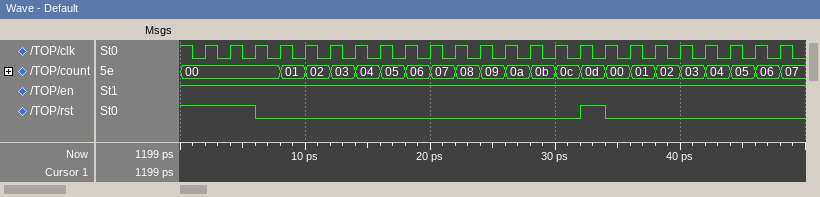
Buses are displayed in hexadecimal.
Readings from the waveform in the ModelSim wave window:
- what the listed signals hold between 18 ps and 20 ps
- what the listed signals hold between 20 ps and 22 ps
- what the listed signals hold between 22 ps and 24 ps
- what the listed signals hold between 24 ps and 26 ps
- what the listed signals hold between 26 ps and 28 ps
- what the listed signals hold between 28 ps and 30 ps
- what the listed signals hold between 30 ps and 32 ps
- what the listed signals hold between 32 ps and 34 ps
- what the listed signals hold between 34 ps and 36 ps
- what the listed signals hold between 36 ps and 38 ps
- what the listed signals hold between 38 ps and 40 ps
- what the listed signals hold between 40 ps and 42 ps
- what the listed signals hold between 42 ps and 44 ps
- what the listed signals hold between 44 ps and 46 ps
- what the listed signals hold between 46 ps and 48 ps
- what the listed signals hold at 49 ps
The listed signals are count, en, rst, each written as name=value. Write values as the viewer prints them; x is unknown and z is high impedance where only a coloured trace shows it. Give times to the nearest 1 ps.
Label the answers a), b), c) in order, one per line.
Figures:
a) count=06, en=1, rst=0
b) count=07, en=1, rst=0
c) count=08, en=1, rst=0
d) count=09, en=1, rst=0
e) count=0a, en=1, rst=0
f) count=0b, en=1, rst=0
g) count=0c, en=1, rst=0
h) count=0d, en=1, rst=1
i) count=00, en=1, rst=0
j) count=01, en=1, rst=0
k) count=02, en=1, rst=0
l) count=03, en=1, rst=0
m) count=04, en=1, rst=0
n) count=05, en=1, rst=0
o) count=06, en=1, rst=0
p) count=07, en=1, rst=0
